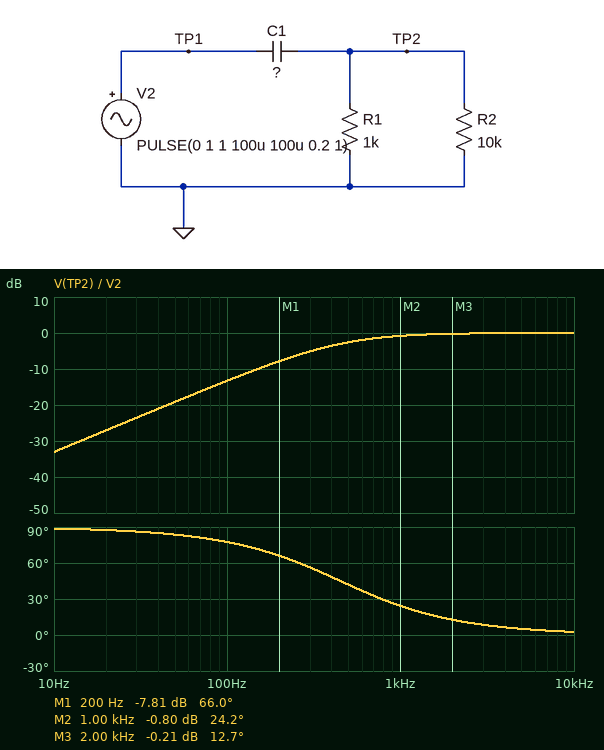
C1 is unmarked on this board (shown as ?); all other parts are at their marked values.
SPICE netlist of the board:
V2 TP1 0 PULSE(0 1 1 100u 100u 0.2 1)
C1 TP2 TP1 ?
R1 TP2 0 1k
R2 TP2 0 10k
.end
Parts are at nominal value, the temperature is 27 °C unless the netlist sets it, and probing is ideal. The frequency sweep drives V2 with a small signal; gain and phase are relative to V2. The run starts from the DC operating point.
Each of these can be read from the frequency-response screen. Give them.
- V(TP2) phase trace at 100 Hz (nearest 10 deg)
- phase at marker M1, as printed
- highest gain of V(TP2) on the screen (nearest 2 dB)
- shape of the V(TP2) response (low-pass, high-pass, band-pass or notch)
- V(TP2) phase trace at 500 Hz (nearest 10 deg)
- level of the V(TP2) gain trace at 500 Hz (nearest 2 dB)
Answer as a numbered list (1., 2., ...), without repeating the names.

1. 80 deg
2. 66.0 deg
3. 0 dB
4. high-pass
5. 40 deg
6. -2 dB
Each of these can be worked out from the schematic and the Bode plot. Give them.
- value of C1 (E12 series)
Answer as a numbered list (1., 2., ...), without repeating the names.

1. 390 nF
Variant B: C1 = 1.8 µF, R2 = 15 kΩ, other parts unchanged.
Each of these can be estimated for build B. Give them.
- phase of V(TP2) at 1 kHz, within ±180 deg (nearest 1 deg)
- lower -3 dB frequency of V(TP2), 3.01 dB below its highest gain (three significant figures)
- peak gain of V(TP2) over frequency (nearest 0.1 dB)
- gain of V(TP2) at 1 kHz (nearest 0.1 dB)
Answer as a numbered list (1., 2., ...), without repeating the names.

1. 5 deg
2. 94.3 Hz
3. 0 dB
4. 0 dB
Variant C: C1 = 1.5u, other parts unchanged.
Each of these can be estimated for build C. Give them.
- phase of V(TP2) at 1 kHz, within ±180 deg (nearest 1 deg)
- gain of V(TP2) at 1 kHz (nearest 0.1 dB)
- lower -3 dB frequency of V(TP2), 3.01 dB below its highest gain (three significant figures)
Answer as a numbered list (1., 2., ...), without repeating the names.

1. 7 deg
2. -0.1 dB
3. 117 Hz
